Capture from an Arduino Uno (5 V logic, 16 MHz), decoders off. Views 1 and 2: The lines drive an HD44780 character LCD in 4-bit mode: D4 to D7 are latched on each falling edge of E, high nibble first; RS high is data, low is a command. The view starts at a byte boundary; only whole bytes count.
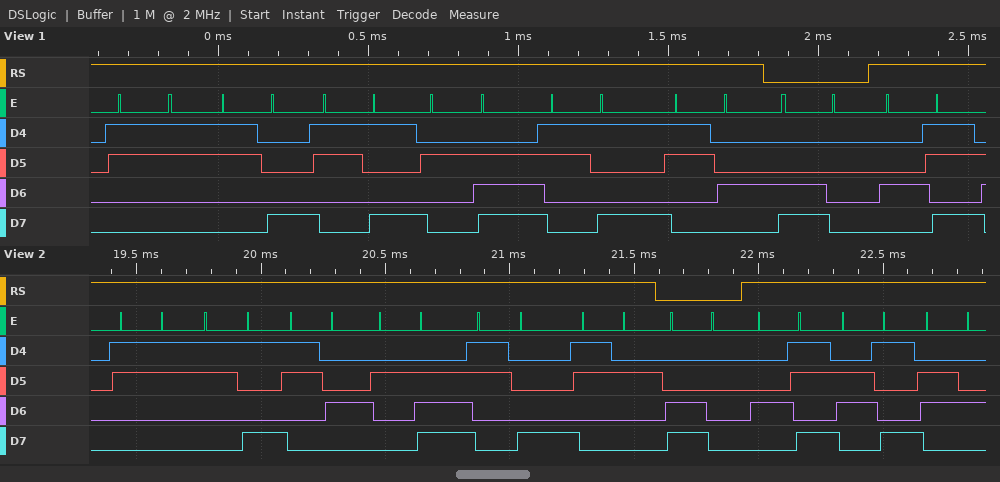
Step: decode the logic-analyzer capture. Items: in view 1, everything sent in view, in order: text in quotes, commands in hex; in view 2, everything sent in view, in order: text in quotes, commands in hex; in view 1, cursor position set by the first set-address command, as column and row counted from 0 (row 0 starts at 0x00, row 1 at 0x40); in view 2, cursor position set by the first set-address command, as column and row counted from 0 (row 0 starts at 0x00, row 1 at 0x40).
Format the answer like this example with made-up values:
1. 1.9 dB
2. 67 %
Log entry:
1. "389.94" 0xC0 "K"
2. "394.82" 0xC0 "Kid"
3. column 0, row 1
4. column 0, row 1
